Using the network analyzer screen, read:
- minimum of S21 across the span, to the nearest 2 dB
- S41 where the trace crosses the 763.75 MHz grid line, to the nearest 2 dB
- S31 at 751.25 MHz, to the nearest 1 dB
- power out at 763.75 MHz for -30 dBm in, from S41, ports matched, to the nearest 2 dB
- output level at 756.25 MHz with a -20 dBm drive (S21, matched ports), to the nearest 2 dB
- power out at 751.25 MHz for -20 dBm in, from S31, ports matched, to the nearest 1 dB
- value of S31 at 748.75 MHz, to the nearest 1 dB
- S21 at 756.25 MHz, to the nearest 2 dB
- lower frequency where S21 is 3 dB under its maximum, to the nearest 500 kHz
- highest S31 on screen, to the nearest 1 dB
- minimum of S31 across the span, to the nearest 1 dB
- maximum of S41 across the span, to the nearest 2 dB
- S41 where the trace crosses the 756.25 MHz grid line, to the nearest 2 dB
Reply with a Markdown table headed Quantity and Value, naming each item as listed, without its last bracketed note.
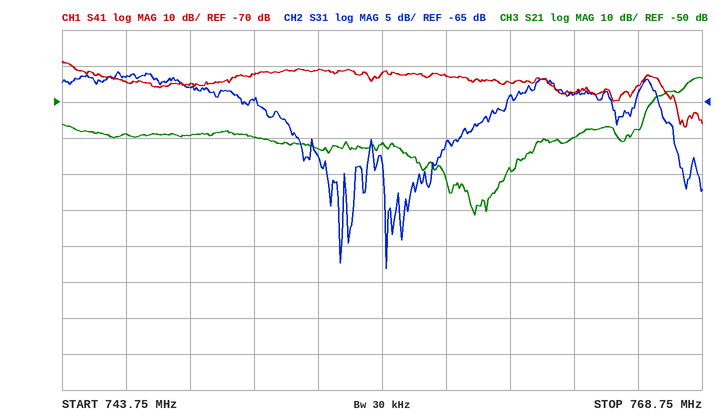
| Quantity | Value |
|---|---|
| minimum of S21 across the span, to the nearest 2 dB | -82 dB |
| S41 where the trace crosses the 763.75 MHz grid line, to the nearest 2 dB | -68 dB |
| S31 at 751.25 MHz, to the nearest 1 dB | -65 dB |
| power out at 763.75 MHz for -30 dBm in, from S41, ports matched, to the nearest 2 dB | -98 dBm |
| output level at 756.25 MHz with a -20 dBm drive (S21, matched ports), to the nearest 2 dB | -82 dBm |
| power out at 751.25 MHz for -20 dBm in, from S31, ports matched, to the nearest 1 dB | -85 dBm |
| value of S31 at 748.75 MHz, to the nearest 1 dB | -63 dB |
| S21 at 756.25 MHz, to the nearest 2 dB | -62 dB |
| lower frequency where S21 is 3 dB under its maximum, to the nearest 500 kHz | 768.0 MHz |
| highest S31 on screen, to the nearest 1 dB | -61 dB |
| minimum of S31 across the span, to the nearest 1 dB | -88 dB |
| maximum of S41 across the span, to the nearest 2 dB | -58 dB |
| S41 where the trace crosses the 756.25 MHz grid line, to the nearest 2 dB | -62 dB |
